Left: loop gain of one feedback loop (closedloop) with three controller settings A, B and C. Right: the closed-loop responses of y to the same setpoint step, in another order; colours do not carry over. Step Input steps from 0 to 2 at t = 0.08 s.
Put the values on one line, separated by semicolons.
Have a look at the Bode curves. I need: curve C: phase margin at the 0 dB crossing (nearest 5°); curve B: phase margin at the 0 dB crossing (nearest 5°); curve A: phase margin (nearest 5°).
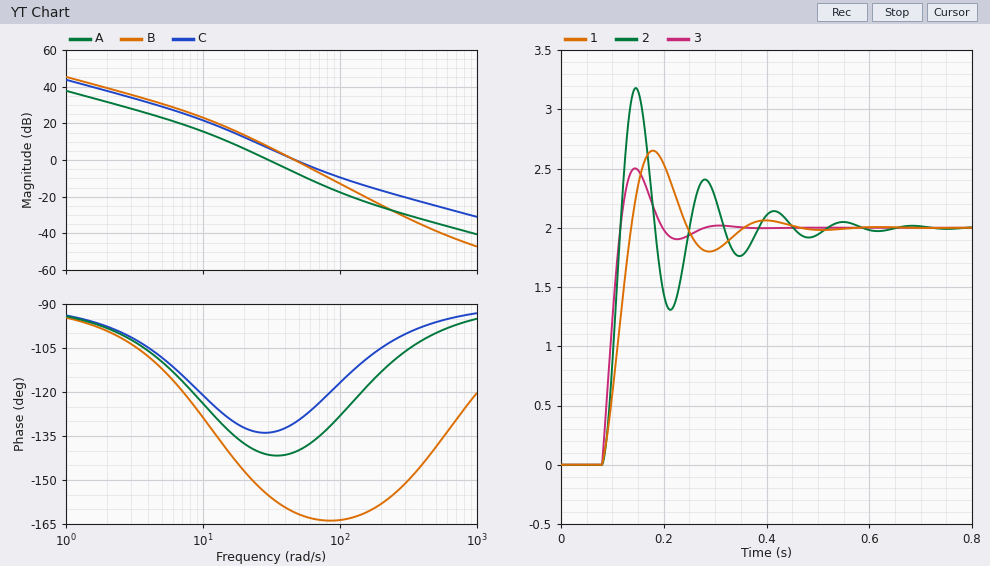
50°; 20°; 40°
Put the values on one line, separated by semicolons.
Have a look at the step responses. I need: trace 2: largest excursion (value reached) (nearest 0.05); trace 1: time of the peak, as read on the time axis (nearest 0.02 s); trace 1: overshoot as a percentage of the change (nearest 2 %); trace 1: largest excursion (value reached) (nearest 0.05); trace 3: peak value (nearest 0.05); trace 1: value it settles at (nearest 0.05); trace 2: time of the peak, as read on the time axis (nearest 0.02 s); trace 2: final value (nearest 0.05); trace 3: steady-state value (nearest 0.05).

3.20; 0.18 s; 32 %; 2.65; 2.50; 2.00; 0.14 s; 2.00; 2.00
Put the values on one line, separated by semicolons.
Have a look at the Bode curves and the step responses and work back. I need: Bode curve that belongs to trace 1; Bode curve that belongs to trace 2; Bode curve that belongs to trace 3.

A; B; C
